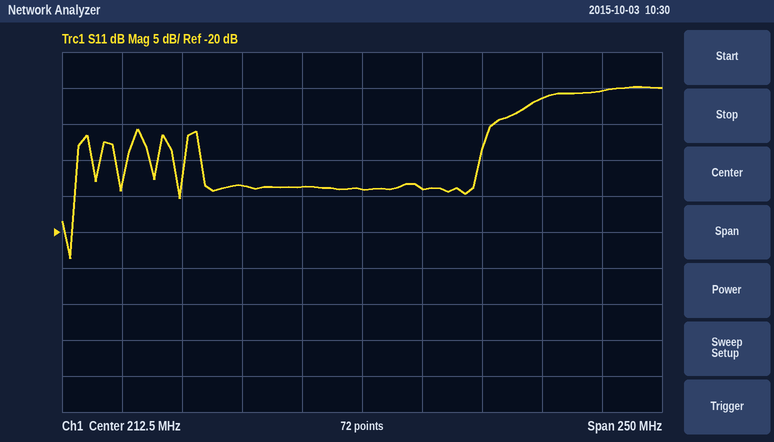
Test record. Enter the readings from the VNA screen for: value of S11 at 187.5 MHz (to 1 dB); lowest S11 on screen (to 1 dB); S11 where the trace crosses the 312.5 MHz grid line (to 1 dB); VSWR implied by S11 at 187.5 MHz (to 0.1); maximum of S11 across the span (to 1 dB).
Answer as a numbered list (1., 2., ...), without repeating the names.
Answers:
1. -14 dB
2. -24 dB
3. 0 dB
4. 1.5
5. 0 dB
